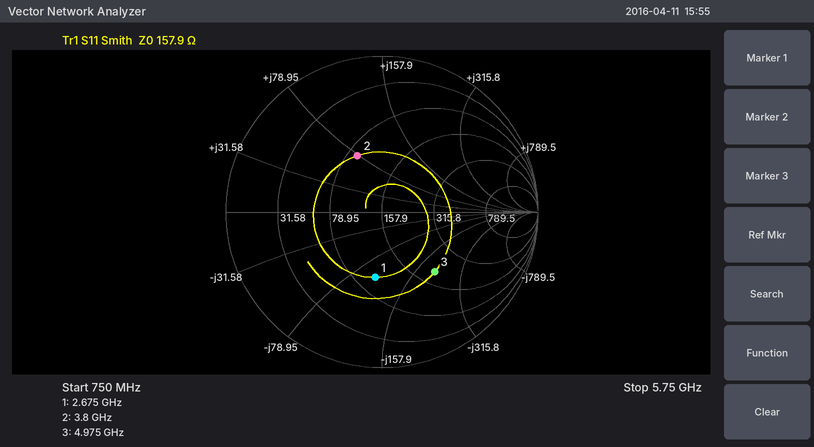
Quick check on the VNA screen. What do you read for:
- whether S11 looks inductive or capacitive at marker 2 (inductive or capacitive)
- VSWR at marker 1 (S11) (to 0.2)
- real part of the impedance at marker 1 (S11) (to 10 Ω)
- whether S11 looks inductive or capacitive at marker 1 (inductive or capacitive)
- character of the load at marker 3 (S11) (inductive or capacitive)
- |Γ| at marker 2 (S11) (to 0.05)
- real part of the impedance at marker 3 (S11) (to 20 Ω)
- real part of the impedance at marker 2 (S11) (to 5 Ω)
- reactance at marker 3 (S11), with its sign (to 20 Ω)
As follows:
inductive
2.4
100 Ω
capacitive
capacitive
0.40
200 Ω
90 Ω
-200 Ω
